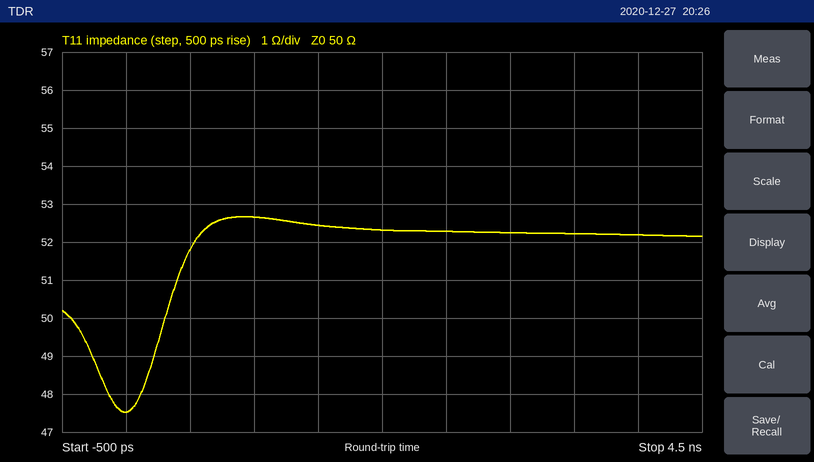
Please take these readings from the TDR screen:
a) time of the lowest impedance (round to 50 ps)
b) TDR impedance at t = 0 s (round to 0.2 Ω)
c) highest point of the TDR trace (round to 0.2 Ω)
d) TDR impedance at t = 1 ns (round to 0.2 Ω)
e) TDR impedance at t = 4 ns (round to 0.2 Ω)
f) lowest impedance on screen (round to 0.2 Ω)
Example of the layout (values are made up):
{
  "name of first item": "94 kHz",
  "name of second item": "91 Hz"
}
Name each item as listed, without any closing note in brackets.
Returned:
{
  "time of the lowest impedance": "0 ps",
  "TDR impedance at t = 0 s": "47.6 Ω",
  "highest point of the TDR trace": "52.6 Ω",
  "TDR impedance at t = 1 ns": "52.6 Ω",
  "TDR impedance at t = 4 ns": "52.2 Ω",
  "lowest impedance on screen": "47.6 Ω"
}
